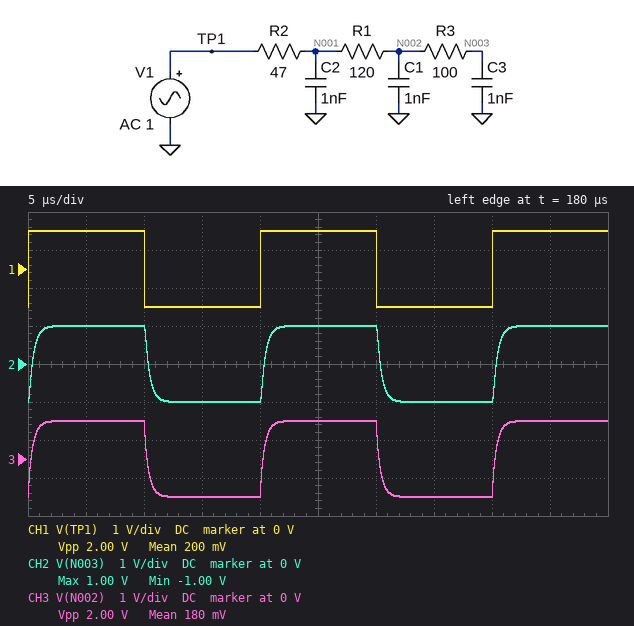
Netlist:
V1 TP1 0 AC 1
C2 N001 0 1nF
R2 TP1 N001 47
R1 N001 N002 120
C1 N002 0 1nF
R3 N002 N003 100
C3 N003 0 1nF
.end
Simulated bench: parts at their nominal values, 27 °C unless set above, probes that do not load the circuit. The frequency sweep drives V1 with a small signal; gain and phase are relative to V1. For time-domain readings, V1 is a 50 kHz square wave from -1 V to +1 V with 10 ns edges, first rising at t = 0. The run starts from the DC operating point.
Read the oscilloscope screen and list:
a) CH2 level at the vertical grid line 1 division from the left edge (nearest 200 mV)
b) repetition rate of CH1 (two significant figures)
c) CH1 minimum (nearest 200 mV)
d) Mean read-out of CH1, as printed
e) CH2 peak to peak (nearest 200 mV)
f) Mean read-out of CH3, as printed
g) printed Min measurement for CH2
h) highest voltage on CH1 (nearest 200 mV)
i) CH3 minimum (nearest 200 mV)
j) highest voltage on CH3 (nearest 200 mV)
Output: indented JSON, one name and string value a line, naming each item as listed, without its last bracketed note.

{
  "CH2 level at the vertical grid line 1 division from the left edge": "1.0 V",
  "repetition rate of CH1": "50 kHz",
  "CH1 minimum": "-1.0 V",
  "Mean read-out of CH1, as printed": "200 mV",
  "CH2 peak to peak": "2.0 V",
  "Mean read-out of CH3, as printed": "180 mV",
  "printed Min measurement for CH2": "-1.00 V",
  "highest voltage on CH1": "1.0 V",
  "CH3 minimum": "-1.0 V",
  "highest voltage on CH3": "1.0 V"
}
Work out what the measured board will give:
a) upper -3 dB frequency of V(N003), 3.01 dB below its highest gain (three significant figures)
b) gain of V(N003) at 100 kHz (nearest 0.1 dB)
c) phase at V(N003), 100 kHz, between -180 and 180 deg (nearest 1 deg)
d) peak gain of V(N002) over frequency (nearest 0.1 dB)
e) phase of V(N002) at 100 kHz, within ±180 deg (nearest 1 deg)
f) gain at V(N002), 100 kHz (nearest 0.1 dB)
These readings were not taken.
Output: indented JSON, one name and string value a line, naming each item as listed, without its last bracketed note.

{
  "upper -3 dB frequency of V(N003), 3.01 dB below its highest gain": "387 kHz",
  "gain of V(N003) at 100 kHz": "-0.3 dB",
  "phase at V(N003), 100 kHz, between -180 and 180 deg": "-17 deg",
  "peak gain of V(N002) over frequency": "0 dB",
  "phase of V(N002) at 100 kHz, within ±180 deg": "-13 deg",
  "gain at V(N002), 100 kHz": "-0.3 dB"
}
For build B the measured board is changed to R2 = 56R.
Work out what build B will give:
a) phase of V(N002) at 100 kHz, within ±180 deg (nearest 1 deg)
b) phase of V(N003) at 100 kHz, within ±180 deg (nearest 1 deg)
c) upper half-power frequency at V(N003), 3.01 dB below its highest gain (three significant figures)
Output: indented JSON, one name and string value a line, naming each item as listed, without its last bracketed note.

{
  "phase of V(N002) at 100 kHz, within ±180 deg": "-14 deg",
  "phase of V(N003) at 100 kHz, within ±180 deg": "-18 deg",
  "upper half-power frequency at V(N003), 3.01 dB below its highest gain": "367 kHz"
}
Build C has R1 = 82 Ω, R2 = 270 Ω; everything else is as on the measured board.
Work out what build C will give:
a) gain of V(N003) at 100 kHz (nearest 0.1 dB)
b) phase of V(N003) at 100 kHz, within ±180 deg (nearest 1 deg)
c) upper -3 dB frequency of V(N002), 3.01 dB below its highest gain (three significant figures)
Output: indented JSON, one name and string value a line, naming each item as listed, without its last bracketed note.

{
  "gain of V(N003) at 100 kHz": "-1.4 dB",
  "phase of V(N003) at 100 kHz, within ±180 deg": "-35 deg",
  "upper -3 dB frequency of V(N002), 3.01 dB below its highest gain": "165 kHz"
}
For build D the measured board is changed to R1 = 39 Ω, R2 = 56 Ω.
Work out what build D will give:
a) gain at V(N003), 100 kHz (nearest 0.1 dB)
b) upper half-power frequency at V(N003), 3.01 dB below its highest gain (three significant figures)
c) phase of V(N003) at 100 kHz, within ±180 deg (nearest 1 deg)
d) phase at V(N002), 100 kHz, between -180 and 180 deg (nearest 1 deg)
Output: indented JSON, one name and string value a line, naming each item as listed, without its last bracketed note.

{
  "gain at V(N003), 100 kHz": "-0.1 dB",
  "upper half-power frequency at V(N003), 3.01 dB below its highest gain": "551 kHz",
  "phase of V(N003) at 100 kHz, within ±180 deg": "-12 deg",
  "phase at V(N002), 100 kHz, between -180 and 180 deg": "-9 deg"
}
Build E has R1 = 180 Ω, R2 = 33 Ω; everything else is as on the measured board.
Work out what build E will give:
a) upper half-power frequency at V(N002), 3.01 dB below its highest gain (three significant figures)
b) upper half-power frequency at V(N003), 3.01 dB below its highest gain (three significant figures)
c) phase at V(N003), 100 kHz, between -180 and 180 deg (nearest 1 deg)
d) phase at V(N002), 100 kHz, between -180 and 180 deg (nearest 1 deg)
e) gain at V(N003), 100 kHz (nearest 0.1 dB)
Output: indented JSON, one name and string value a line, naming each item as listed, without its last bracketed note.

{
  "upper half-power frequency at V(N002), 3.01 dB below its highest gain": "337 kHz",
  "upper half-power frequency at V(N003), 3.01 dB below its highest gain": "323 kHz",
  "phase at V(N003), 100 kHz, between -180 and 180 deg": "-20 deg",
  "phase at V(N002), 100 kHz, between -180 and 180 deg": "-16 deg",
  "gain at V(N003), 100 kHz": "-0.4 dB"
}
